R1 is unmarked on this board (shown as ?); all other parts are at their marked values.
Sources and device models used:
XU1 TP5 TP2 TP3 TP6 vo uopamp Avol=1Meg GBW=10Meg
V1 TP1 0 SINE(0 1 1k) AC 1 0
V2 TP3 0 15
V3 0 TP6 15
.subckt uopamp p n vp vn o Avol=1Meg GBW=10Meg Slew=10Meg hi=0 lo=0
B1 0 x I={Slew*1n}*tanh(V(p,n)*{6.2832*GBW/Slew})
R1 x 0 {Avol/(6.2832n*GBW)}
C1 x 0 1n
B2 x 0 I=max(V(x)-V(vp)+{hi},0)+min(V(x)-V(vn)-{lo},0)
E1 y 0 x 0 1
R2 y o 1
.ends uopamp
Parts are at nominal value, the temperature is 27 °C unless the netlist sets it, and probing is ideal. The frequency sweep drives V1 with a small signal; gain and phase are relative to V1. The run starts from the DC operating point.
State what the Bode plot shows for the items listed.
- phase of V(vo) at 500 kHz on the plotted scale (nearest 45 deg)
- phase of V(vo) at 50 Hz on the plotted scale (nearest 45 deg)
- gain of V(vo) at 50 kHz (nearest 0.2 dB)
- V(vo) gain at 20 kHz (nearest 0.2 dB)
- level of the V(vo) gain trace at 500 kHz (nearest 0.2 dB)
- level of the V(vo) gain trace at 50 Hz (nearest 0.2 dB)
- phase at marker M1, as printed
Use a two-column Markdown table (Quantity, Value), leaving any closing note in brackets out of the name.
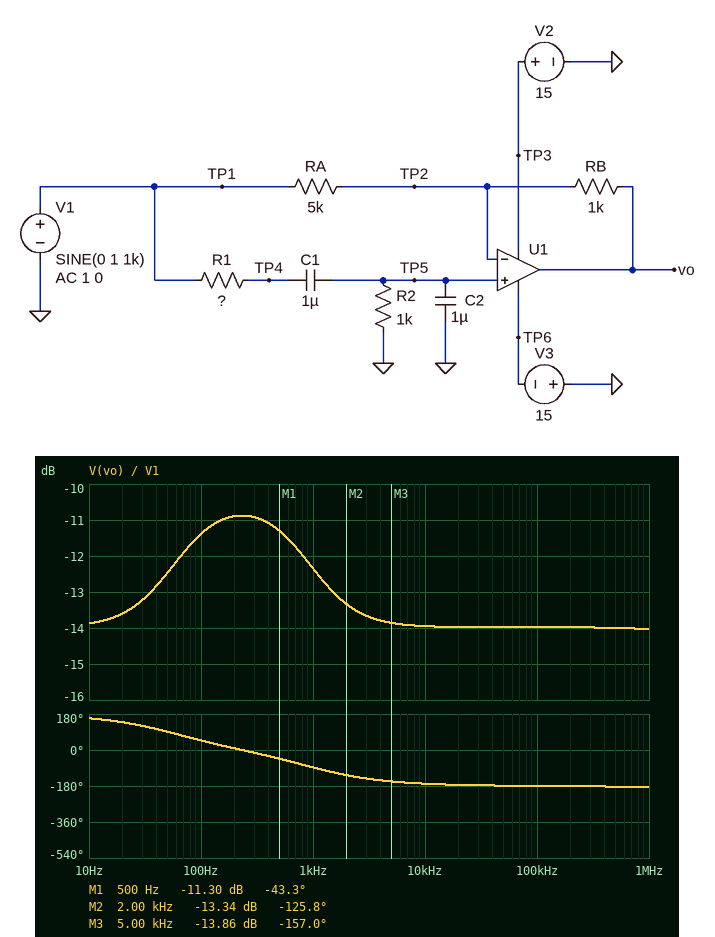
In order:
| Quantity | Value |
|---|---|
| phase of V(vo) at 500 kHz on the plotted scale | -180 deg |
| phase of V(vo) at 50 Hz on the plotted scale | 90 deg |
| gain of V(vo) at 50 kHz | -14.0 dB |
| V(vo) gain at 20 kHz | -14.0 dB |
| level of the V(vo) gain trace at 500 kHz | -14.0 dB |
| level of the V(vo) gain trace at 50 Hz | -12.4 dB |
| phase at marker M1, as printed | -43.3 deg |
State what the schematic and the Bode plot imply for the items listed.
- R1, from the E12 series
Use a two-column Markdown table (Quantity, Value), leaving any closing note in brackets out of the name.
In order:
| Quantity | Value |
|---|---|
| R1, from the E12 series | 470 Ω |
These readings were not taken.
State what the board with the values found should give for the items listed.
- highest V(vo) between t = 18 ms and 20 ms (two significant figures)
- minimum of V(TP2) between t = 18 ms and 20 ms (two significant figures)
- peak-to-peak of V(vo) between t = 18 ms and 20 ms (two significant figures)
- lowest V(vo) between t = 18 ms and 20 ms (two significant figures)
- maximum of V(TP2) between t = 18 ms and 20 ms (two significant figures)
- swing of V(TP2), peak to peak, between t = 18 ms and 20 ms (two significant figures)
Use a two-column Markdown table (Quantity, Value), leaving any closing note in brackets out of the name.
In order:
| Quantity | Value |
|---|---|
| highest V(vo) between t = 18 ms and 20 ms | 240 mV |
| minimum of V(TP2) between t = 18 ms and 20 ms | -270 mV |
| peak-to-peak of V(vo) between t = 18 ms and 20 ms | 480 mV |
| lowest V(vo) between t = 18 ms and 20 ms | -240 mV |
| maximum of V(TP2) between t = 18 ms and 20 ms | 270 mV |
| swing of V(TP2), peak to peak, between t = 18 ms and 20 ms | 540 mV |
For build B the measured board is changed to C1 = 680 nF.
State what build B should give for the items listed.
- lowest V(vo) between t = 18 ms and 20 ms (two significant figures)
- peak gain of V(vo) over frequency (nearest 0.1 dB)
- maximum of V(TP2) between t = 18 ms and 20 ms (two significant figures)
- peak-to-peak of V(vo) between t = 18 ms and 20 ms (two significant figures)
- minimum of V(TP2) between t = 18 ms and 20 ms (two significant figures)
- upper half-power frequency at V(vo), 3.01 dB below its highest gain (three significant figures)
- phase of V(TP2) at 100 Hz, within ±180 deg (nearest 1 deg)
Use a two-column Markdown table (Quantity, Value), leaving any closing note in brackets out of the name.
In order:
| Quantity | Value |
|---|---|
| lowest V(vo) between t = 18 ms and 20 ms | -200 mV |
| peak gain of V(vo) over frequency | -13.6 dB |
| maximum of V(TP2) between t = 18 ms and 20 ms | 250 mV |
| peak-to-peak of V(vo) between t = 18 ms and 20 ms | 410 mV |
| minimum of V(TP2) between t = 18 ms and 20 ms | -250 mV |
| upper half-power frequency at V(vo), 3.01 dB below its highest gain | 7.67 MHz |
| phase of V(TP2) at 100 Hz, within ±180 deg | 35 deg |
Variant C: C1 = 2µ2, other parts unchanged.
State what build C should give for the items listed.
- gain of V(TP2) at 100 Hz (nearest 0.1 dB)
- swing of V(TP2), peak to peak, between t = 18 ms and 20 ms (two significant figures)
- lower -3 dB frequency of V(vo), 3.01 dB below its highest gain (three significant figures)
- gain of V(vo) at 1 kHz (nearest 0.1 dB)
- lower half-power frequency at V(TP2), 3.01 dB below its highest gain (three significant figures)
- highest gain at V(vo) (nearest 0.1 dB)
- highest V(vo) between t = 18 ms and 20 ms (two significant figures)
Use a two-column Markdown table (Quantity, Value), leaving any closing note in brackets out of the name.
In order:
| Quantity | Value |
|---|---|
| gain of V(TP2) at 100 Hz | -5.9 dB |
| swing of V(TP2), peak to peak, between t = 18 ms and 20 ms | 580 mV |
| lower -3 dB frequency of V(vo), 3.01 dB below its highest gain | 27.1 Hz |
| gain of V(vo) at 1 kHz | -10.8 dB |
| lower half-power frequency at V(TP2), 3.01 dB below its highest gain | 35.6 Hz |
| highest gain at V(vo) | -7.5 dB |
| highest V(vo) between t = 18 ms and 20 ms | 290 mV |
